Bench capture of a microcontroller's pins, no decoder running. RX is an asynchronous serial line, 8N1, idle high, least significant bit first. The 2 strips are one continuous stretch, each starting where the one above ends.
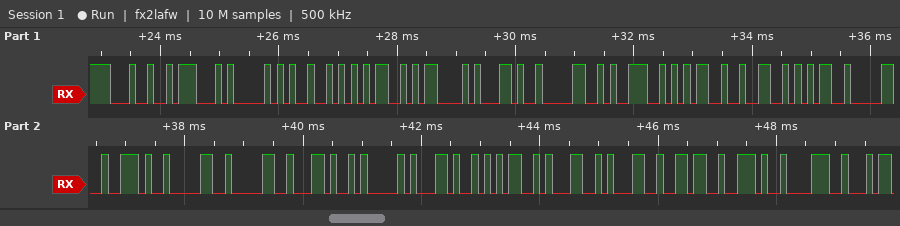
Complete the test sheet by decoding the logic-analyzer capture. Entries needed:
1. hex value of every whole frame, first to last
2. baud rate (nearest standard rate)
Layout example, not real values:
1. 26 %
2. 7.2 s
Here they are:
1. 24 47 50 52 4D 43 2C 30 39 35 32 35 30 2E 30 30 2C 41 2C 35 31 31 36 2E 38
2. 9600 baud
